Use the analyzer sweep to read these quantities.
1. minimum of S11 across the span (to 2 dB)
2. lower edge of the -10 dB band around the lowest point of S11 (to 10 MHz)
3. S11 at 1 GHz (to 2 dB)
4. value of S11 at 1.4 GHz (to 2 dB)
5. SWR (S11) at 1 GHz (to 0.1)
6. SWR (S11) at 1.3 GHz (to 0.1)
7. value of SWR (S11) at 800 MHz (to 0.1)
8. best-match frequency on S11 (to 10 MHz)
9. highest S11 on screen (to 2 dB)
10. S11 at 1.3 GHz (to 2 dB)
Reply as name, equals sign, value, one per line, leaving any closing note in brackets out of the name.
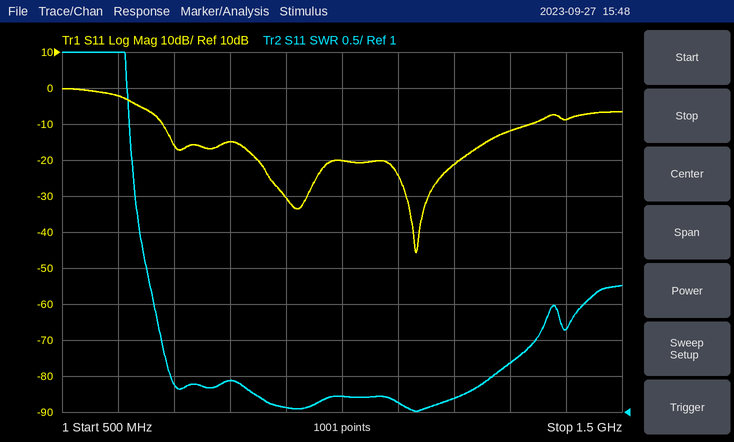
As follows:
minimum of S11 across the span = -46 dB
lower edge of the -10 dB band around the lowest point of S11 = 680 MHz
S11 at 1 GHz = -20 dB
value of S11 at 1.4 GHz = -8 dB
SWR (S11) at 1 GHz = 1.2
SWR (S11) at 1.3 GHz = 1.7
value of SWR (S11) at 800 MHz = 1.4
best-match frequency on S11 = 1.13 GHz
highest S11 on screen = 0 dB
S11 at 1.3 GHz = -12 dB
